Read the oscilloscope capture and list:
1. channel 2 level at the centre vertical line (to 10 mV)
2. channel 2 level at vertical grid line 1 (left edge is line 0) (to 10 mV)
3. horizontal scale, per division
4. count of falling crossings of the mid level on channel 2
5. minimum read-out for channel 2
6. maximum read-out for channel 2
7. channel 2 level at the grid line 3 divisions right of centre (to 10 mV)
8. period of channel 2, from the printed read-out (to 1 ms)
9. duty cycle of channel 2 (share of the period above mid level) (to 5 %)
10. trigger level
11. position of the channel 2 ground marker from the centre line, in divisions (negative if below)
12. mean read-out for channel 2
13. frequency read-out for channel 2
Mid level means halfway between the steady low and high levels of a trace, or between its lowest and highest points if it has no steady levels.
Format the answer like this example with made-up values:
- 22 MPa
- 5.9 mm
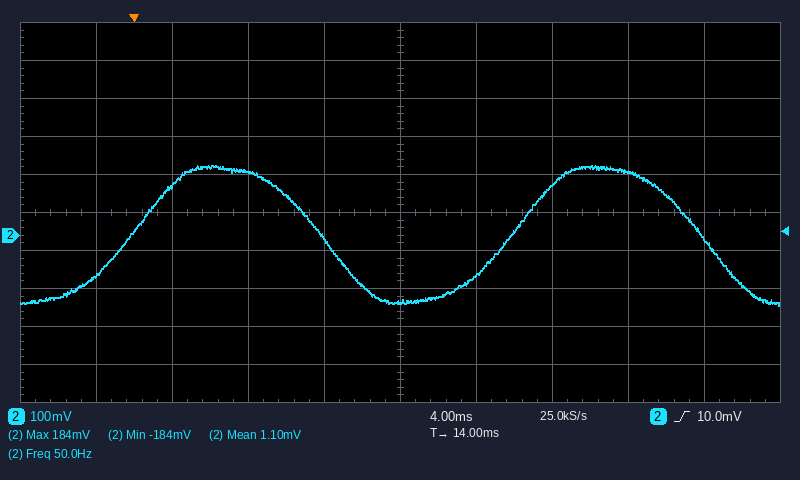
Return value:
- -170 mV
- -110 mV
- 4 ms
- 2
- -184 mV
- 184 mV
- 170 mV
- 20 ms
- 50 %
- 10.0 mV
- -0.6 div
- 1.10 mV
- 50.0 Hz
